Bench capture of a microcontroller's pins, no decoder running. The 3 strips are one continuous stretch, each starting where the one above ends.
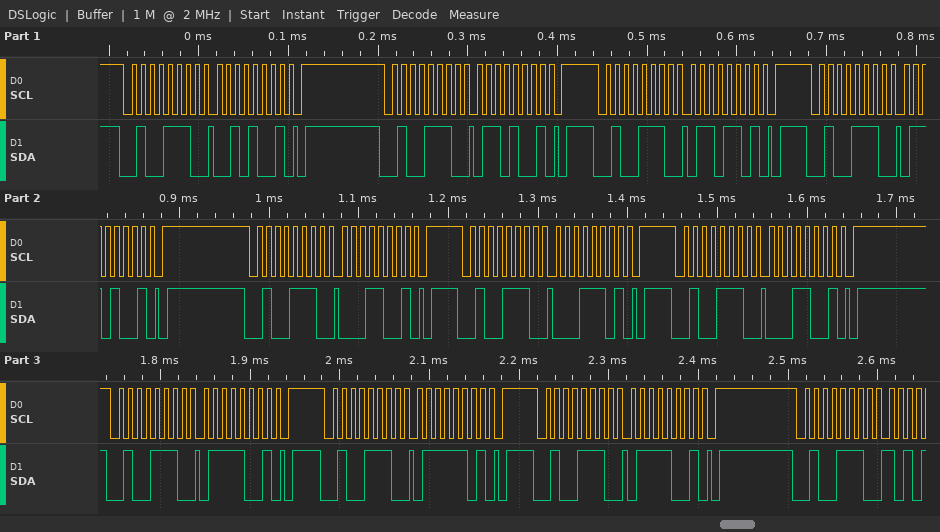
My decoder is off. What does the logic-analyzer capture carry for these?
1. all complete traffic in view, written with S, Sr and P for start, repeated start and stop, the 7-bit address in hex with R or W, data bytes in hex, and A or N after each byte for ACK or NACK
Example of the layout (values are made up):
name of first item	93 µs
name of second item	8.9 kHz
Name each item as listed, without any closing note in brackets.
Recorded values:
all complete traffic in view, written with S, Sr and P for start, repeated start and stop, the 7-bit address in hex with R or W, data bytes in hex, and A or N after each byte for ACK or NACK	S 27W A 29 A P S 27W A 69 A P S 27W A 6D A P S 27W A 69 A P S 27W A 19 A P S 27W A 1D A P S 27W A 19 A P S 27W A 79 A P S 27W A 7D A P S 27W A 79 A P S 27W A
